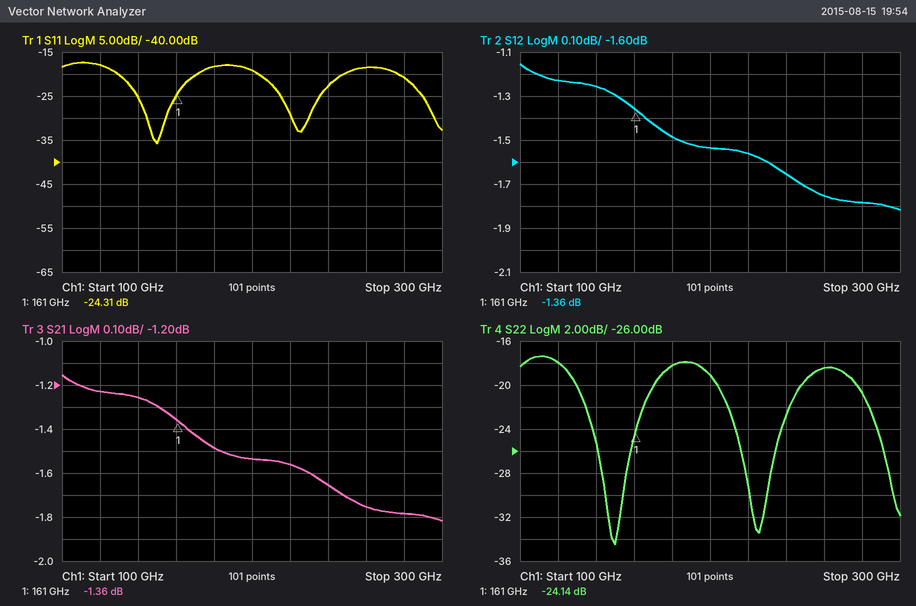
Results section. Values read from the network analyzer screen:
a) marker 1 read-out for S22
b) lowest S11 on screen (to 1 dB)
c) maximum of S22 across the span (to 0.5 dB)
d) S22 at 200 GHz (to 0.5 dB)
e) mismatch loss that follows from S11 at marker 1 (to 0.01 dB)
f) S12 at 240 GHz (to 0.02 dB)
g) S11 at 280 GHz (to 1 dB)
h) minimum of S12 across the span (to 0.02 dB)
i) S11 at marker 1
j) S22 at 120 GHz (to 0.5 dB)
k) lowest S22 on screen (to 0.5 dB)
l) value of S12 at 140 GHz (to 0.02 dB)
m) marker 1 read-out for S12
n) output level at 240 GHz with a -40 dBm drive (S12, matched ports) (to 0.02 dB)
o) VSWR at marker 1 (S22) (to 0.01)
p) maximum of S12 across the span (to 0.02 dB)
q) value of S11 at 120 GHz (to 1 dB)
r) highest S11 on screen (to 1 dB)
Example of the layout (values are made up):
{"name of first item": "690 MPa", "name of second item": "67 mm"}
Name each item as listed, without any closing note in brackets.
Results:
{"marker 1 read-out for S22": "-24.14 dB", "lowest S11 on screen": "-36 dB", "maximum of S22 across the span": "-17.5 dB", "S22 at 200 GHz": "-19.0 dB", "mismatch loss that follows from S11 at marker 1": "0.02 dB", "S12 at 240 GHz": "-1.66 dB", "S11 at 280 GHz": "-21 dB", "minimum of S12 across the span": "-1.82 dB", "S11 at marker 1": "-24.31 dB", "S22 at 120 GHz": "-18.0 dB", "lowest S22 on screen": "-34.5 dB", "value of S12 at 140 GHz": "-1.26 dB", "marker 1 read-out for S12": "-1.36 dB", "output level at 240 GHz with a -40 dBm drive (S12, matched ports)": "-41.66 dBm", "VSWR at marker 1 (S22)": "1.13", "maximum of S12 across the span": "-1.16 dB", "value of S11 at 120 GHz": "-18 dB", "highest S11 on screen": "-17 dB"}
